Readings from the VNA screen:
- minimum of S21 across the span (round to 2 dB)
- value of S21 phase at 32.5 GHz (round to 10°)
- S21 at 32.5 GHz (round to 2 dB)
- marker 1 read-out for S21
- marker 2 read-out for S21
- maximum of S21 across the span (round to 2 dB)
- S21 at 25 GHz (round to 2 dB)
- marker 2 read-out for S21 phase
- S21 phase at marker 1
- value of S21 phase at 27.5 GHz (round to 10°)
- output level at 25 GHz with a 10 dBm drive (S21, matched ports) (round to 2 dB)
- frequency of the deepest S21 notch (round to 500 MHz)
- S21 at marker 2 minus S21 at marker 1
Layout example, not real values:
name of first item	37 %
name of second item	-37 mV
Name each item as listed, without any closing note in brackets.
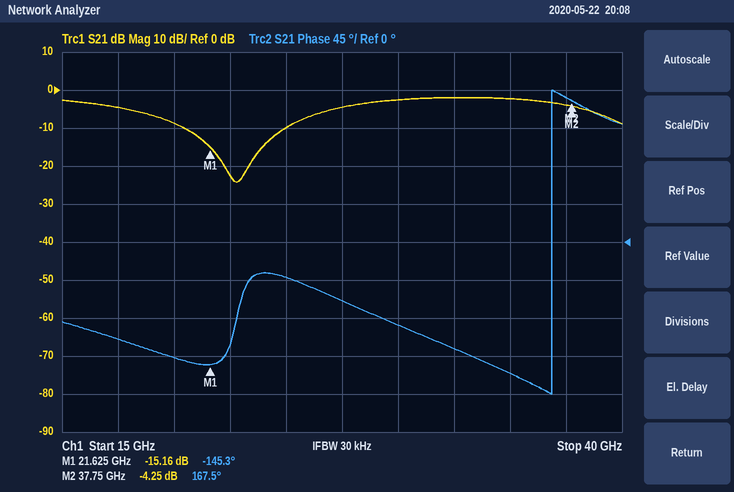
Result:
minimum of S21 across the span	-24 dB
value of S21 phase at 32.5 GHz	-130°
S21 at 32.5 GHz	-2 dB
marker 1 read-out for S21	-15.16 dB
marker 2 read-out for S21	-4.25 dB
maximum of S21 across the span	-2 dB
S21 at 25 GHz	-10 dB
marker 2 read-out for S21 phase	167.5°
S21 phase at marker 1	-145.3°
value of S21 phase at 27.5 GHz	-70°
output level at 25 GHz with a 10 dBm drive (S21, matched ports)	0 dBm
frequency of the deepest S21 notch	23.0 GHz
S21 at marker 2 minus S21 at marker 1	10.91 dB
